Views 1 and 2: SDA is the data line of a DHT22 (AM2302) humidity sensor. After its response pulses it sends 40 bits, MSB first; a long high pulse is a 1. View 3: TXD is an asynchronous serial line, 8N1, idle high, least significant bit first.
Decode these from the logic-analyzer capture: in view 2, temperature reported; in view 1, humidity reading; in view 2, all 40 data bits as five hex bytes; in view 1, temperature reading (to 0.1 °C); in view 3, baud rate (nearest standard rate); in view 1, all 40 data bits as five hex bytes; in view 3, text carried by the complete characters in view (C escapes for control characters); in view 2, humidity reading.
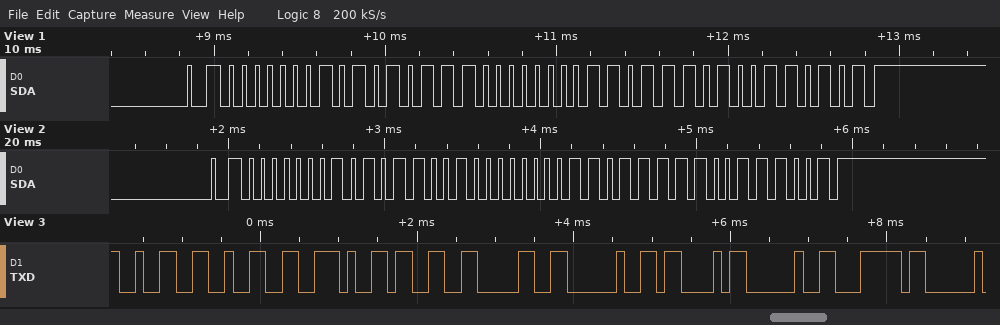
22.3 °C
34.3 %
01 59 00 DF 39
22.1 °C
9600 baud
01 57 00 DD 35
"22.30 C |"
34.5 %
